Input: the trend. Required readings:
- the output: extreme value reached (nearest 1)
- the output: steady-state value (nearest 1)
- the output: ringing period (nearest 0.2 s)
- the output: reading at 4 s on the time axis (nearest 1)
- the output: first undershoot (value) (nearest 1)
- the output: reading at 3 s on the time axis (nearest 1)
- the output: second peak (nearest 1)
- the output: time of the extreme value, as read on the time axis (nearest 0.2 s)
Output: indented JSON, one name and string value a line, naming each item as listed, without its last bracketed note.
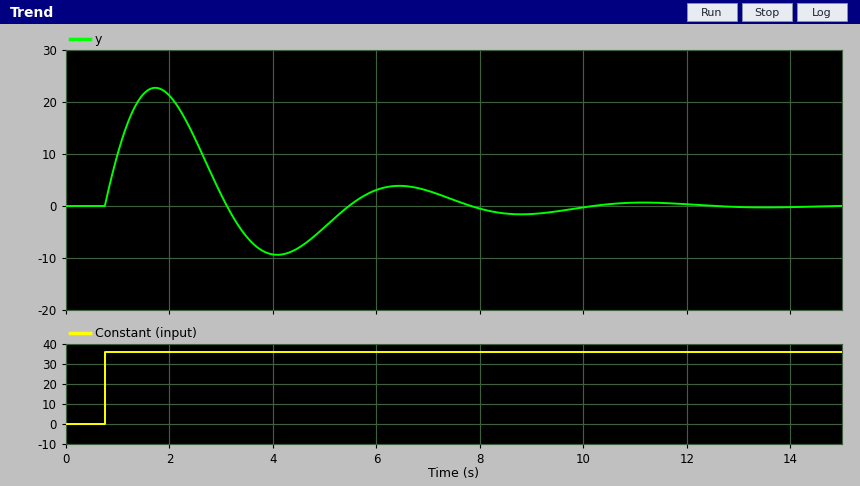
{
  "the output: extreme value reached": "23",
  "the output: steady-state value": "0",
  "the output: ringing period": "4.8 s",
  "the output: reading at 4 s on the time axis": "-9",
  "the output: first undershoot (value)": "-9",
  "the output: reading at 3 s on the time axis": "2",
  "the output: second peak": "4",
  "the output: time of the extreme value, as read on the time axis": "1.8 s"
}
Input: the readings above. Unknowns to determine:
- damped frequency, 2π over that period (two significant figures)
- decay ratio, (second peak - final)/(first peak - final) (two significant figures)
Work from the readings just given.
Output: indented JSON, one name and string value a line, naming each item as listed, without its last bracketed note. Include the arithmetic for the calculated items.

{
  "damped frequency, 2π over that period": "2π / 4.8 = 1.3 rad/s",
  "decay ratio, (second peak - final)/(first peak - final)": "(4 - 0) / (23 - 0) = 0.17"
}
